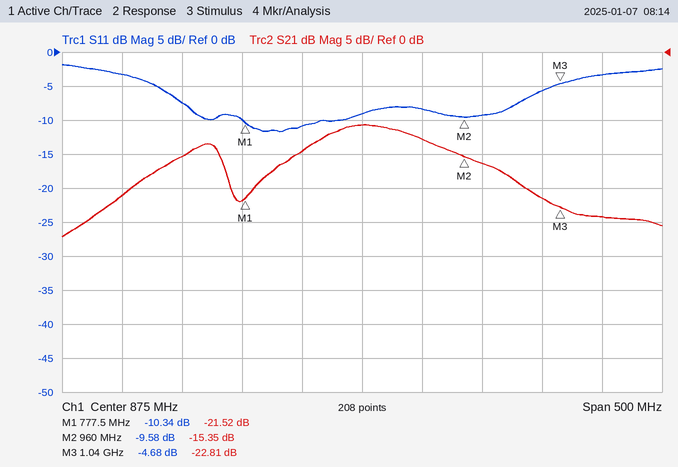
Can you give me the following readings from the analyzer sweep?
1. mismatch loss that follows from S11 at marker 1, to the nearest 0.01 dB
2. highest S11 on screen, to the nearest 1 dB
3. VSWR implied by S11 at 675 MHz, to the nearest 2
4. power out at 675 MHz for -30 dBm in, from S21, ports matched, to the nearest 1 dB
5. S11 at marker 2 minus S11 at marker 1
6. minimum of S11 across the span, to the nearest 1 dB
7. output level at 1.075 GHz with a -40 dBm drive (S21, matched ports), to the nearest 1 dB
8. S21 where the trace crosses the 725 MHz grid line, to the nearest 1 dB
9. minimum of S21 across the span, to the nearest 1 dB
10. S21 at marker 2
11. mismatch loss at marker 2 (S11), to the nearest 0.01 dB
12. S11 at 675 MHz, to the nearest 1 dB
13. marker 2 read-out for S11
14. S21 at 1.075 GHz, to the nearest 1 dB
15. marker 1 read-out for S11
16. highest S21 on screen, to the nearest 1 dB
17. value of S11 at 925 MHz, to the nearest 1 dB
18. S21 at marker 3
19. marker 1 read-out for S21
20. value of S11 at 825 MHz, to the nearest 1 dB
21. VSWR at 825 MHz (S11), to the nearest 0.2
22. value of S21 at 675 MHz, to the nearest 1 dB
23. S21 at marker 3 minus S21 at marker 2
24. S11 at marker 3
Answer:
0.42 dB
-2 dB
6
-51 dBm
0.76 dB
-12 dB
-64 dBm
-15 dB
-27 dB
-15.35 dB
0.51 dB
-3 dB
-9.58 dB
-24 dB
-10.34 dB
-11 dB
-8 dB
-22.81 dB
-21.52 dB
-11 dB
1.8
-21 dB
-7.46 dB
-4.68 dB
